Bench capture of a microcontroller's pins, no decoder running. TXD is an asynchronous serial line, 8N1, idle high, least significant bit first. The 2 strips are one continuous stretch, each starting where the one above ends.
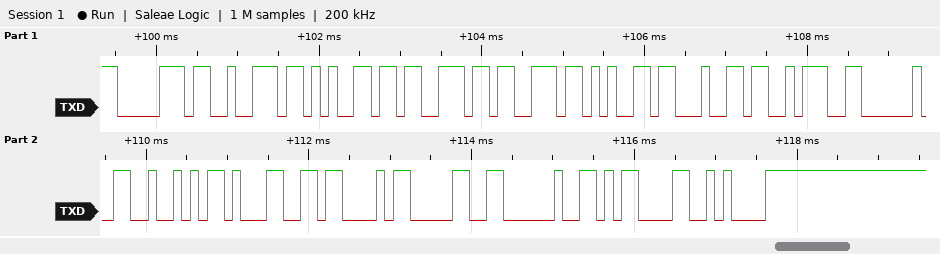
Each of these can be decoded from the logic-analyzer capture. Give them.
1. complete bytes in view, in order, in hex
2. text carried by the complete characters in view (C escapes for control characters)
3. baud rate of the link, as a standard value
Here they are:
70 72 65 73 73 65 64 3A 20 52 31 43 30 20 0D 0A
"pressed: R1C0 \r\n"
9600 baud
